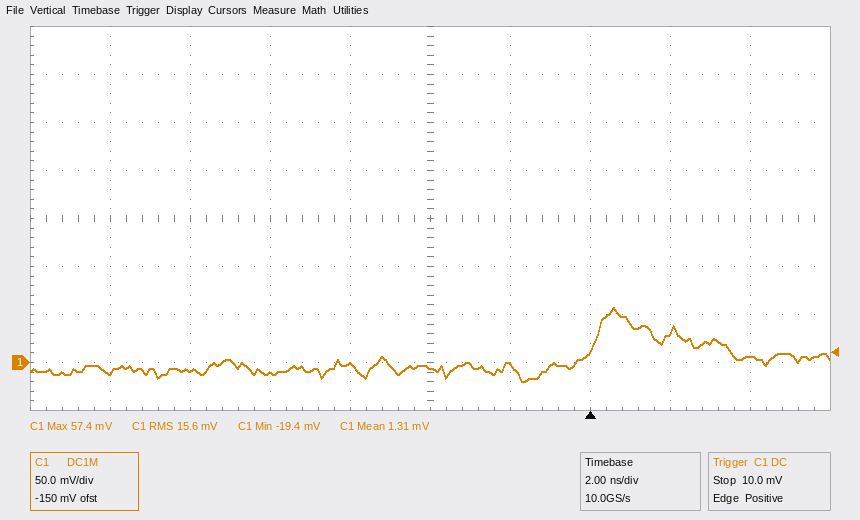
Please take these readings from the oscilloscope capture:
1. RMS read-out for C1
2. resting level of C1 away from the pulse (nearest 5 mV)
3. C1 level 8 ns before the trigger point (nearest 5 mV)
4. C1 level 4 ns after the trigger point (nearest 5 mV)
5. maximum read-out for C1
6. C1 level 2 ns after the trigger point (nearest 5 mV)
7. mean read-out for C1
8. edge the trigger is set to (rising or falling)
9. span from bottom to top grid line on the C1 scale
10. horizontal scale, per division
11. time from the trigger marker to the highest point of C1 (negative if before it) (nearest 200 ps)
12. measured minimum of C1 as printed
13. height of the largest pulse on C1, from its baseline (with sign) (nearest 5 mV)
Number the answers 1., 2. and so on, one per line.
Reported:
1. 15.6 mV
2. -5 mV
3. -10 mV
4. 5 mV
5. 57.4 mV
6. 35 mV
7. 1.31 mV
8. rising
9. 400 mV
10. 2 ns
11. +600 ps
12. -19.4 mV
13. +65 mV
